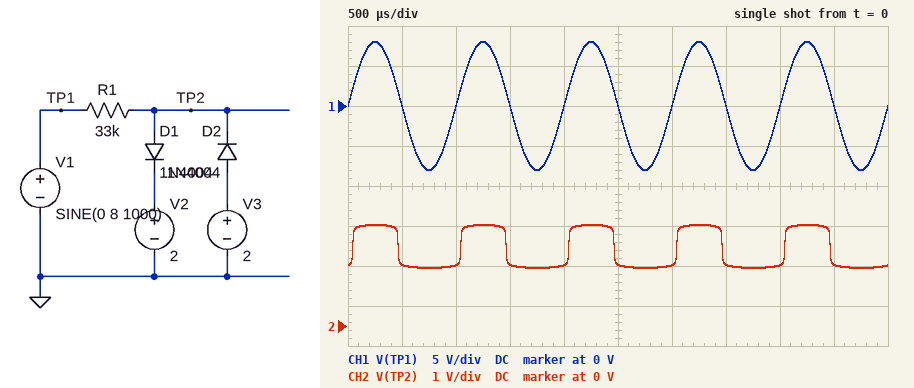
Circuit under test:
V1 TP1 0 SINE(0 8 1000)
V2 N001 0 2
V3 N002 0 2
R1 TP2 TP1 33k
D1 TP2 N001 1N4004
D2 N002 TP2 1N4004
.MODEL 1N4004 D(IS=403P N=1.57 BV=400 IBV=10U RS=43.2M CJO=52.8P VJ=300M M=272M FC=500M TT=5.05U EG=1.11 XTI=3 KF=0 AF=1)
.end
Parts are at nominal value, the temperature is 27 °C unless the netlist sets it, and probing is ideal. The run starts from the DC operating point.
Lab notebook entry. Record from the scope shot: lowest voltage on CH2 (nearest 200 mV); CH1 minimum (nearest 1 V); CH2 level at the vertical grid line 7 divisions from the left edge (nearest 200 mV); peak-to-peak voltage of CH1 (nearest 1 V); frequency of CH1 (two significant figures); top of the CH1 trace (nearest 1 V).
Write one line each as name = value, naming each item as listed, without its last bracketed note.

lowest voltage on CH2 = 1.4 V
CH1 minimum = -8 V
CH2 level at the vertical grid line 7 divisions from the left edge = 1.6 V
peak-to-peak voltage of CH1 = 16 V
frequency of CH1 = 1.0 kHz
top of the CH1 trace = 8 V
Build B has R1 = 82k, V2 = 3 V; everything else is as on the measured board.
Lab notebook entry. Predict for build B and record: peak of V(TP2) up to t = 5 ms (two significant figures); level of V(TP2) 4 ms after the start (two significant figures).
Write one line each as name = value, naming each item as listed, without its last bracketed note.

peak of V(TP2) up to t = 5 ms = 3.5 V
level of V(TP2) 4 ms after the start = 1.6 V
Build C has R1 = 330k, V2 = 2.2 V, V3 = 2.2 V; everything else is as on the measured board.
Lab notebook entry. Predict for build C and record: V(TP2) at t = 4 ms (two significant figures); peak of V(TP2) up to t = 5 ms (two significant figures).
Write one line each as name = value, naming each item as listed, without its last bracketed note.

V(TP2) at t = 4 ms = 1.8 V
peak of V(TP2) up to t = 5 ms = 2.6 V
